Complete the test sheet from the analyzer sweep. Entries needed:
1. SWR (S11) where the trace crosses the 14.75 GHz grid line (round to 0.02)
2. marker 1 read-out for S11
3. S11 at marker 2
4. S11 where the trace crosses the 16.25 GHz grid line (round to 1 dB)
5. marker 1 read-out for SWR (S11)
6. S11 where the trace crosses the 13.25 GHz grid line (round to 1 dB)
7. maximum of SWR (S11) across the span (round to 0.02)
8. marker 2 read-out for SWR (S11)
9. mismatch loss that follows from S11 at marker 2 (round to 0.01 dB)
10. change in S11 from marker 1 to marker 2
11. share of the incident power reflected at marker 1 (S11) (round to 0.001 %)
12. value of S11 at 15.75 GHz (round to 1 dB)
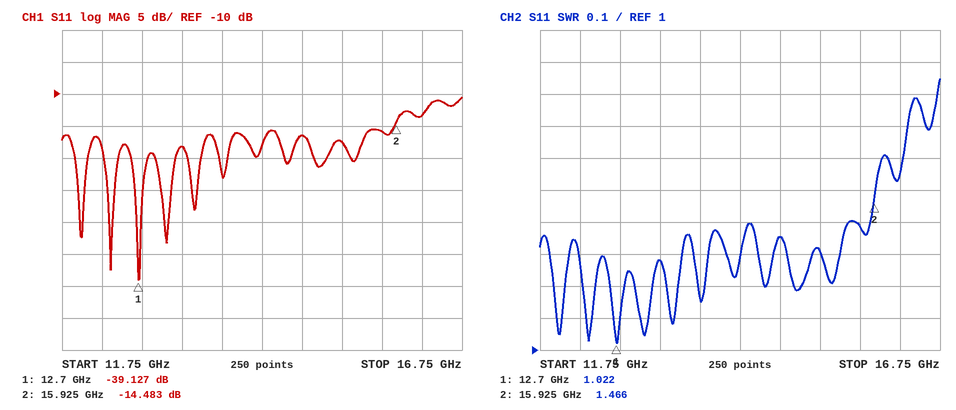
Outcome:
1.36
-39.127 dB
-14.483 dB
-13 dB
1.022
-18 dB
1.84
1.466
0.16 dB
24.644 dB
0.012 %
-16 dB
